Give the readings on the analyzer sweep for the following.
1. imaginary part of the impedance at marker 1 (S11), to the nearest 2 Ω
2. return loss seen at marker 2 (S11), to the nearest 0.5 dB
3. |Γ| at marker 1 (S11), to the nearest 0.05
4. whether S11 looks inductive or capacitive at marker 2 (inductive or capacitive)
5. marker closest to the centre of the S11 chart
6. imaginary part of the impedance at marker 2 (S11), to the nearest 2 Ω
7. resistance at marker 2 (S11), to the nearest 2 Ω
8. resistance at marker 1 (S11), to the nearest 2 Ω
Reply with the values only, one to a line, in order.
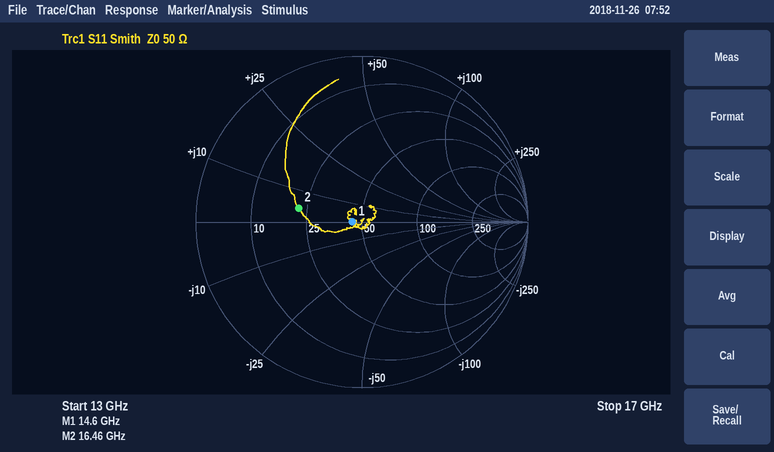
0 Ω
8.0 dB
0.05
inductive
marker 1
+4 Ω
22 Ω
44 Ω
